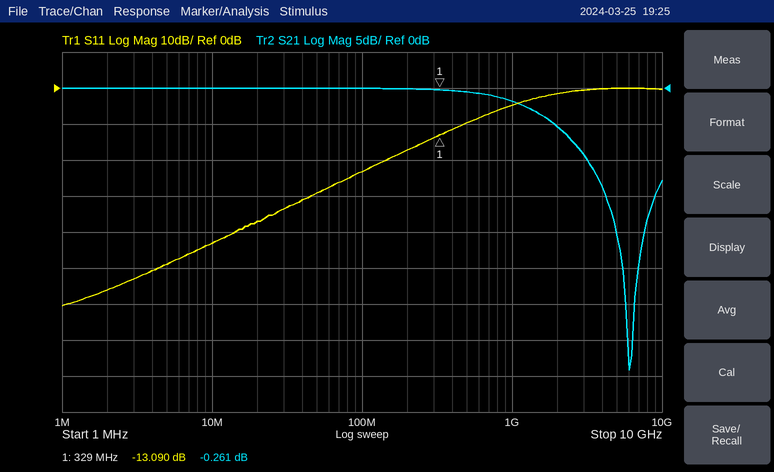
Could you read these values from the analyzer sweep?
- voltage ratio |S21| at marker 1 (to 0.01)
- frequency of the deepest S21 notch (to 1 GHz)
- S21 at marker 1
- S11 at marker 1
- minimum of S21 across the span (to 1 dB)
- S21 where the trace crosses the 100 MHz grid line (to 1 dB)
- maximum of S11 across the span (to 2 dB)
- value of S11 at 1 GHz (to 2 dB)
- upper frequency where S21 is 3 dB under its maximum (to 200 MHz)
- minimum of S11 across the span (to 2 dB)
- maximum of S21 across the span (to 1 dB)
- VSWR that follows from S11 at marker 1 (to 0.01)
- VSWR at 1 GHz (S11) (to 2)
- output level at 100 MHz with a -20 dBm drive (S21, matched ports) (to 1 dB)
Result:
0.97
6 GHz
-0.261 dB
-13.090 dB
-39 dB
0 dB
0 dB
-4 dB
1.4 GHz
-60 dB
0 dB
1.57
4
-20 dBm
